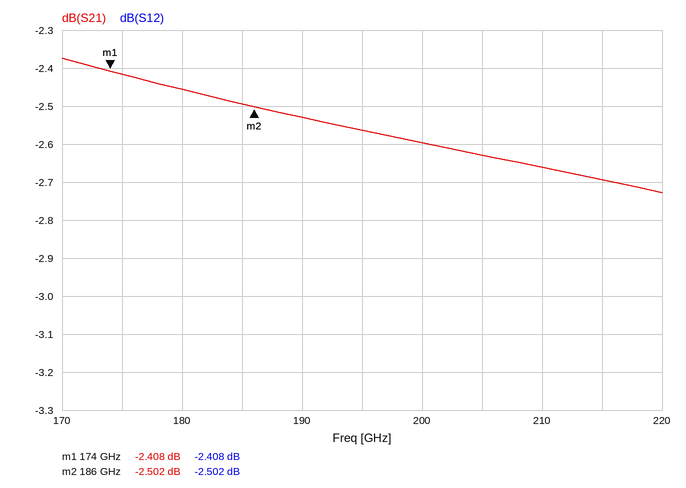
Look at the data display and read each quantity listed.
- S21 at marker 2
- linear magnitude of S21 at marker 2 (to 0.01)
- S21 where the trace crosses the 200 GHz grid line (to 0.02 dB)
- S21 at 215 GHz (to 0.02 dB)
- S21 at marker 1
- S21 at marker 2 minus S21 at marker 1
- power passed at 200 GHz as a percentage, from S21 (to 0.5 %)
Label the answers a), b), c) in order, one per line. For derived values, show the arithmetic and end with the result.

a) -2.502 dB
b) 10^(-2.502/20) ≈ 0.75
c) -2.60 dB
d) -2.70 dB
e) -2.408 dB
f) -2.502 − (-2.408) = -0.094 dB
g) 10^(-2.6/10) ≈ 55.0 %
